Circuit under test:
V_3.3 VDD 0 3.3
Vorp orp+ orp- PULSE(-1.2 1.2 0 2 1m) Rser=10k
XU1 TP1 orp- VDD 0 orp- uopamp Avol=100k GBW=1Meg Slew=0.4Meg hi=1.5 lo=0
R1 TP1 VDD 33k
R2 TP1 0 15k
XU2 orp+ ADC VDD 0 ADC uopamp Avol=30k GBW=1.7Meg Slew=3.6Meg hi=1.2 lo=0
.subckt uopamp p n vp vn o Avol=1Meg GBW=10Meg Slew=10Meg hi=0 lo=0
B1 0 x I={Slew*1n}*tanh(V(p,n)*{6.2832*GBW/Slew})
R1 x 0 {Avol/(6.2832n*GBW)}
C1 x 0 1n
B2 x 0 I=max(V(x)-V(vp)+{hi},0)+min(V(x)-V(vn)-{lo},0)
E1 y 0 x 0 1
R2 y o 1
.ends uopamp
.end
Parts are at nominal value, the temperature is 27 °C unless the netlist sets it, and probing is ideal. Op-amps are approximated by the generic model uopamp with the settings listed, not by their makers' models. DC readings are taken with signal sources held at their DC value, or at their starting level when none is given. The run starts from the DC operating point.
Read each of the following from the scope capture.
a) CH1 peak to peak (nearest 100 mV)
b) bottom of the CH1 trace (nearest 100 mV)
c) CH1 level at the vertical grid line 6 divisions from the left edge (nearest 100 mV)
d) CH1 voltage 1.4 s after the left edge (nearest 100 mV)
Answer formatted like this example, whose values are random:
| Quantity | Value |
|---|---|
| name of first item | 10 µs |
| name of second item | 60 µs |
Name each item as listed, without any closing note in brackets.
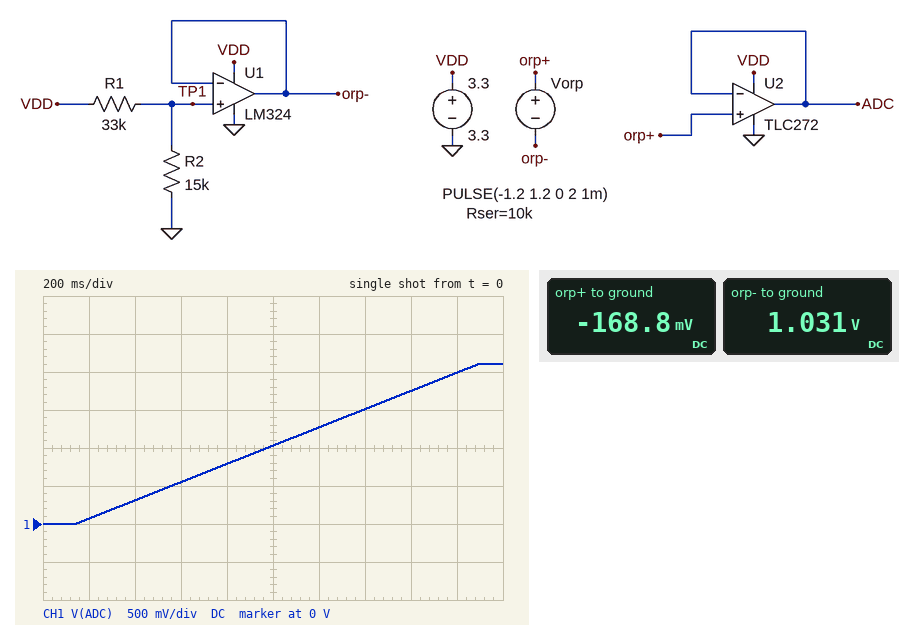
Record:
| Quantity | Value |
|---|---|
| CH1 peak to peak | 2.1 V |
| bottom of the CH1 trace | 0 V |
| CH1 level at the vertical grid line 6 divisions from the left edge | 1.3 V |
| CH1 voltage 1.4 s after the left edge | 1.5 V |
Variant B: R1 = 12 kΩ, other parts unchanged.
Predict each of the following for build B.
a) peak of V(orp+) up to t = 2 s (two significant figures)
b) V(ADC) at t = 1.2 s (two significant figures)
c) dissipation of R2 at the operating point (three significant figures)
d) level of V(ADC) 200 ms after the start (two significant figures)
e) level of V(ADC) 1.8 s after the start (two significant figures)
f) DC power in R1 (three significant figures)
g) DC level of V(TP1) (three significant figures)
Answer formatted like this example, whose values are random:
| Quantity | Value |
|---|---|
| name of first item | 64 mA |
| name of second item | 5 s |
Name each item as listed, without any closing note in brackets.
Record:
| Quantity | Value |
|---|---|
| peak of V(orp+) up to t = 2 s | 3.0 V |
| V(ADC) at t = 1.2 s | 2.0 V |
| dissipation of R2 at the operating point | 224 µW |
| level of V(ADC) 200 ms after the start | 840 mV |
| level of V(ADC) 1.8 s after the start | 2.1 V |
| DC power in R1 | 179 µW |
| DC level of V(TP1) | 1.83 V |
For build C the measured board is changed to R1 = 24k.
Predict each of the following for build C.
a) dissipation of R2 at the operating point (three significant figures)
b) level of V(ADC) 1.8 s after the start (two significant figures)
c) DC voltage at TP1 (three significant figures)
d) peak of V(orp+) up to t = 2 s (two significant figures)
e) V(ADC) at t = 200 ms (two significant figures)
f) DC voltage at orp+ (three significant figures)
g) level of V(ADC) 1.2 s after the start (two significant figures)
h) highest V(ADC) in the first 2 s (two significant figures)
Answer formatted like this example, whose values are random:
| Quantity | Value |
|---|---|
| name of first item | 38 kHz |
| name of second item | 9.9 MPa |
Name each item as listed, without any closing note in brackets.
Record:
| Quantity | Value |
|---|---|
| dissipation of R2 at the operating point | 107 µW |
| level of V(ADC) 1.8 s after the start | 2.1 V |
| DC voltage at TP1 | 1.27 V |
| peak of V(orp+) up to t = 2 s | 2.5 V |
| V(ADC) at t = 200 ms | 310 mV |
| DC voltage at orp+ | 69.2 mV |
| level of V(ADC) 1.2 s after the start | 1.5 V |
| highest V(ADC) in the first 2 s | 2.1 V |
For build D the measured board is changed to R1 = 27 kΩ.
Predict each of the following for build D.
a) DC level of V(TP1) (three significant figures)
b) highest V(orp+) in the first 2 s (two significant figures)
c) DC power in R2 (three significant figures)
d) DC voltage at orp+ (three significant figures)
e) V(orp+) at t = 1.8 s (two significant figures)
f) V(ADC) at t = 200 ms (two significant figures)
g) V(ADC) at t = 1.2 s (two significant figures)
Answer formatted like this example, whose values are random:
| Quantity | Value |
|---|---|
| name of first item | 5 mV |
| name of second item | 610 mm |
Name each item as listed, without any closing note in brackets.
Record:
| Quantity | Value |
|---|---|
| DC level of V(TP1) | 1.18 V |
| highest V(orp+) in the first 2 s | 2.4 V |
| DC power in R2 | 92.6 µW |
| DC voltage at orp+ | -21.4 mV |
| V(orp+) at t = 1.8 s | 2.1 V |
| V(ADC) at t = 200 ms | 220 mV |
| V(ADC) at t = 1.2 s | 1.4 V |
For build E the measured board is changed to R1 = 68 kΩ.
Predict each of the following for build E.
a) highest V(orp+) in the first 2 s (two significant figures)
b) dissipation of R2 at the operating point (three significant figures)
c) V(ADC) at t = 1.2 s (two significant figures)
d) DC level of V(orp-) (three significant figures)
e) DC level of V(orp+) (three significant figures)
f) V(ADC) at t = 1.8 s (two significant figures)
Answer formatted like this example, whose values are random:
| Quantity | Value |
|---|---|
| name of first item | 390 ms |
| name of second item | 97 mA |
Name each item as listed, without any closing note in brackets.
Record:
| Quantity | Value |
|---|---|
| highest V(orp+) in the first 2 s | 1.8 V |
| dissipation of R2 at the operating point | 23.7 µW |
| V(ADC) at t = 1.2 s | 840 mV |
| DC level of V(orp-) | 596 mV |
| DC level of V(orp+) | -604 mV |
| V(ADC) at t = 1.8 s | 1.6 V |
